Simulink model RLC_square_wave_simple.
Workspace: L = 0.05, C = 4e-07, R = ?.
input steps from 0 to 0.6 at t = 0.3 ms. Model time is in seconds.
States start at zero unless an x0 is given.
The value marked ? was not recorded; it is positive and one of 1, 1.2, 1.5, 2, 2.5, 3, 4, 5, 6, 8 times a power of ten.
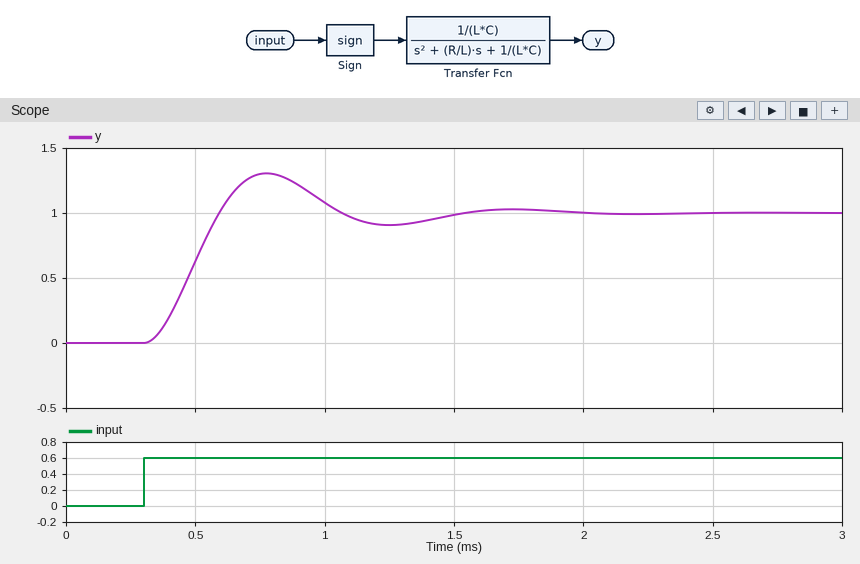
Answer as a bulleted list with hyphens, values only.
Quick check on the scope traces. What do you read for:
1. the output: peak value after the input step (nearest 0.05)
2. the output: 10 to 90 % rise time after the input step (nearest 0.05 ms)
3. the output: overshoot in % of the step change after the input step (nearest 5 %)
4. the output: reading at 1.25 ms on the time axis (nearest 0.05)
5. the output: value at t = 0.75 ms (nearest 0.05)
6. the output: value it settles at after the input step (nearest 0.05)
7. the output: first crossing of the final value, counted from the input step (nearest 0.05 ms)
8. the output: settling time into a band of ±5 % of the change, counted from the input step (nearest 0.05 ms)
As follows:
- 1.30
- 0.20 ms
- 30 %
- 0.90
- 1.30
- 1.00
- 0.30 ms
- 1.10 ms
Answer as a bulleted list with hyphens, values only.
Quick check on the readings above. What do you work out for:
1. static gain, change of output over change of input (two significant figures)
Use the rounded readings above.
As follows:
- 1.7
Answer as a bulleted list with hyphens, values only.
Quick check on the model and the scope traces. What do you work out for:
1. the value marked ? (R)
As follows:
- 250
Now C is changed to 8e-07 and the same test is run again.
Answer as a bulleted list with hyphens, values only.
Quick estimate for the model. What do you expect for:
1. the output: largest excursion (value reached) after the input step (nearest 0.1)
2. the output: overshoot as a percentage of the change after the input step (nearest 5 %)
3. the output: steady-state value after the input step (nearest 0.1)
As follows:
- 1.2
- 15 %
- 1.0
